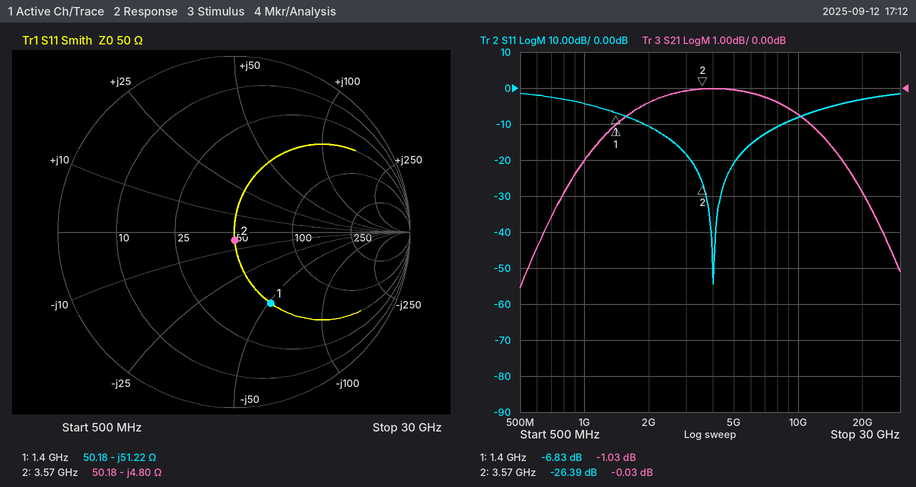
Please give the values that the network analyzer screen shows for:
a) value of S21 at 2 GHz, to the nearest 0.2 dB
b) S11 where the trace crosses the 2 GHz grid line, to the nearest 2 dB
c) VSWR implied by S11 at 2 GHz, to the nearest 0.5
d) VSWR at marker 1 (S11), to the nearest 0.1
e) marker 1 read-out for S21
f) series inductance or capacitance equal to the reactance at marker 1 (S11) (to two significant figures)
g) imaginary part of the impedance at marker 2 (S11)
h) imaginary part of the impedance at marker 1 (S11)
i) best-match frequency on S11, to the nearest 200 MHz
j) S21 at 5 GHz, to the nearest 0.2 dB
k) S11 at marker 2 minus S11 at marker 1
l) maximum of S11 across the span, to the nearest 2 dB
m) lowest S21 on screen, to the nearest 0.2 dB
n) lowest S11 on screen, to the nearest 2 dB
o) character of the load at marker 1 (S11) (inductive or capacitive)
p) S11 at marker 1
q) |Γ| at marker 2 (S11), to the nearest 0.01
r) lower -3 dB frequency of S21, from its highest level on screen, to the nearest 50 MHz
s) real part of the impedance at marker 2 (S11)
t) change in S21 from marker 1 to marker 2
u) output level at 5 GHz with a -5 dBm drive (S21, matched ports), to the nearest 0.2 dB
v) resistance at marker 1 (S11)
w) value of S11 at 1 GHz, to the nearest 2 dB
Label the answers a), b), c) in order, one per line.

a) -0.4 dB
b) -10 dB
c) 2.0
d) 2.7
e) -1.03 dB
f) 2.2 pF
g) -4.80 Ω
h) -51.22 Ω
i) 4.0 GHz
j) 0.0 dB
k) -19.56 dB
l) -2 dB
m) -5.6 dB
n) -54 dB
o) capacitive
p) -6.83 dB
q) 0.05
r) 800 MHz
s) 50.18 Ω
t) 1.00 dB
u) -5.0 dBm
v) 50.18 Ω
w) -4 dB
